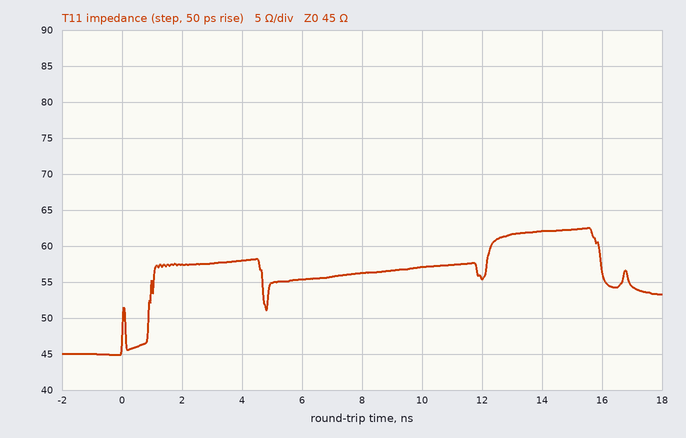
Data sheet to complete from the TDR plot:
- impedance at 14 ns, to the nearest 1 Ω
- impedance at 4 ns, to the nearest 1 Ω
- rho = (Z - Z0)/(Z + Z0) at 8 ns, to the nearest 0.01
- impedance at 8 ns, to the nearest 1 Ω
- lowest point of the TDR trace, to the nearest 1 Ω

62 Ω
58 Ω
+0.11
56 Ω
45 Ω
